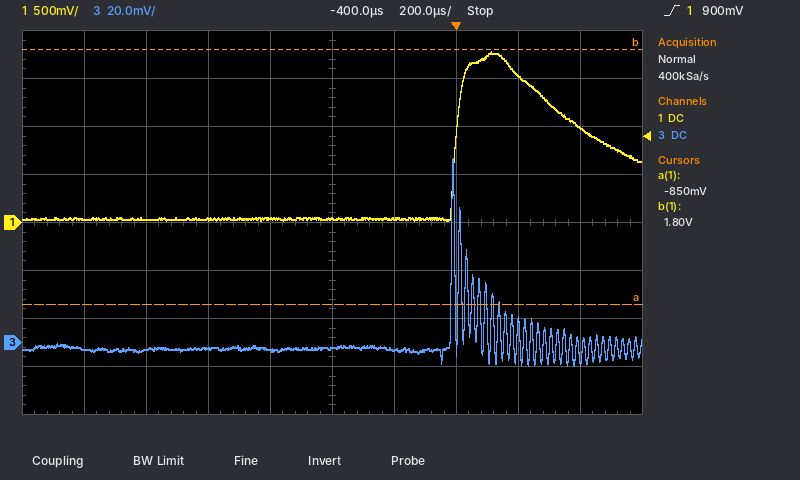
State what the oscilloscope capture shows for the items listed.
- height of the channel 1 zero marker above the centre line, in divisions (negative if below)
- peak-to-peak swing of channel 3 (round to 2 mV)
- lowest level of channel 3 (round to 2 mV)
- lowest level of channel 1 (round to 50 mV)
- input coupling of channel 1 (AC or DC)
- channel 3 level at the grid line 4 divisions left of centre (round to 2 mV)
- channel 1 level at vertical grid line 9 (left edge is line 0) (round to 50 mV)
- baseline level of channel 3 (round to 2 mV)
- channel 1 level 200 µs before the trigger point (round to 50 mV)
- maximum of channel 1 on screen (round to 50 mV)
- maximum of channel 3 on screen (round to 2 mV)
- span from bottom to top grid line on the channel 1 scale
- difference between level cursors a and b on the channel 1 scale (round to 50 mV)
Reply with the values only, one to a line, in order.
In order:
0.0 div
86 mV
-10 mV
0 mV
DC
-2 mV
1.00 V
-2 mV
50 mV
1.80 V
76 mV
4 V
2.65 V
